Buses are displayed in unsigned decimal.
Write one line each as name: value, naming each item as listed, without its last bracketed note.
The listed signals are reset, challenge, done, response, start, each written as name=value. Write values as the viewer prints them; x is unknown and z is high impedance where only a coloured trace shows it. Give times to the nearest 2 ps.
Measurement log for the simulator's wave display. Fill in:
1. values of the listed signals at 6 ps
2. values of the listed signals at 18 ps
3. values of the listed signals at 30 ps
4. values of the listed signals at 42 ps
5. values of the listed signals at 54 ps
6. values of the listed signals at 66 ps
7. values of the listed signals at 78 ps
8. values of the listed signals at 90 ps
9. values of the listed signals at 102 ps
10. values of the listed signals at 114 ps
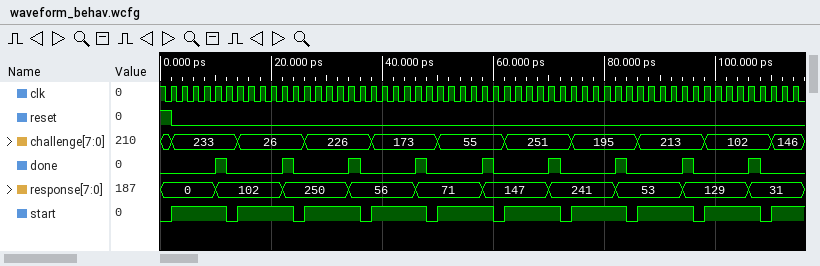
values of the listed signals at 6 ps: reset=0, challenge=233, done=0, response=0, start=1
values of the listed signals at 18 ps: reset=0, challenge=26, done=0, response=102, start=1
values of the listed signals at 30 ps: reset=0, challenge=226, done=0, response=250, start=1
values of the listed signals at 42 ps: reset=0, challenge=173, done=0, response=56, start=1
values of the listed signals at 54 ps: reset=0, challenge=55, done=0, response=71, start=1
values of the listed signals at 66 ps: reset=0, challenge=251, done=0, response=147, start=1
values of the listed signals at 78 ps: reset=0, challenge=195, done=0, response=241, start=1
values of the listed signals at 90 ps: reset=0, challenge=213, done=0, response=53, start=1
values of the listed signals at 102 ps: reset=0, challenge=102, done=0, response=129, start=1
values of the listed signals at 114 ps: reset=0, challenge=146, done=0, response=31, start=1
